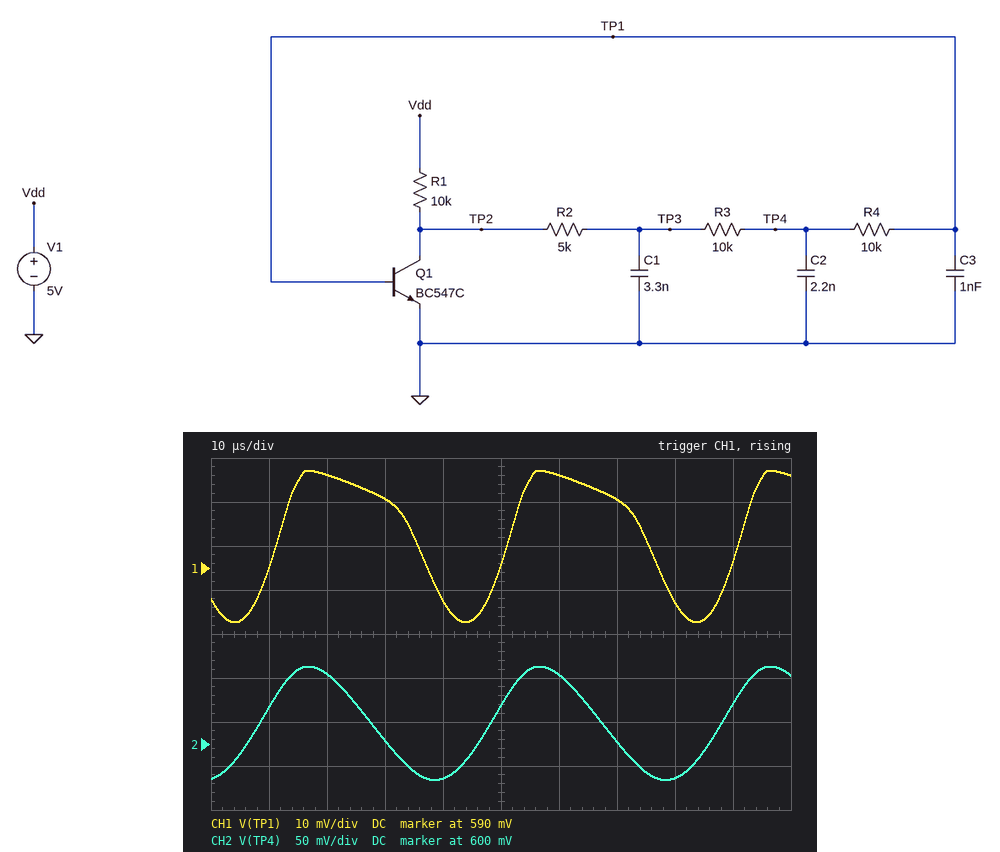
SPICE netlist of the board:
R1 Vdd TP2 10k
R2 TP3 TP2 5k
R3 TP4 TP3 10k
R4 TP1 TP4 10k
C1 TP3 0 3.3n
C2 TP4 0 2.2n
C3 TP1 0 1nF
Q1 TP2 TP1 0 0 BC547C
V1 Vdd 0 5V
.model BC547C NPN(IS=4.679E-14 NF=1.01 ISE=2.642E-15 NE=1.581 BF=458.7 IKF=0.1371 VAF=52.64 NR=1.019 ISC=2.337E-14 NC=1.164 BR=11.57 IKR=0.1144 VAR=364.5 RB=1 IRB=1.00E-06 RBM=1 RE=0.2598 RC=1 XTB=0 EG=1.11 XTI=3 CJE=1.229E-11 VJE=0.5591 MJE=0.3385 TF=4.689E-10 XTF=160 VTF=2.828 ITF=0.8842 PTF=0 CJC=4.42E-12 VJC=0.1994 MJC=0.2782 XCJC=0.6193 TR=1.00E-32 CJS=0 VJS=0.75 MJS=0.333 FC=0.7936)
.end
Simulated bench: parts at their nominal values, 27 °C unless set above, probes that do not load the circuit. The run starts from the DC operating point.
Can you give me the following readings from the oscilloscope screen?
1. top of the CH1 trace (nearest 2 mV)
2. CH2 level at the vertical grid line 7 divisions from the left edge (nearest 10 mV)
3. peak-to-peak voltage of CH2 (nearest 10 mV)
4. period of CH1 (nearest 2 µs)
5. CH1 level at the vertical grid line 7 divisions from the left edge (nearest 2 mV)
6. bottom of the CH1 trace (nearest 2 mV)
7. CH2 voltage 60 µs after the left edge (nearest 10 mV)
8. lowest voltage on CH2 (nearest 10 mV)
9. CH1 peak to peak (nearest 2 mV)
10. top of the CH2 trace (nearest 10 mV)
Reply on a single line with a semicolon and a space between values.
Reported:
612 mV; 600 mV; 130 mV; 40 µs; 606 mV; 578 mV; 680 mV; 560 mV; 34 mV; 690 mV
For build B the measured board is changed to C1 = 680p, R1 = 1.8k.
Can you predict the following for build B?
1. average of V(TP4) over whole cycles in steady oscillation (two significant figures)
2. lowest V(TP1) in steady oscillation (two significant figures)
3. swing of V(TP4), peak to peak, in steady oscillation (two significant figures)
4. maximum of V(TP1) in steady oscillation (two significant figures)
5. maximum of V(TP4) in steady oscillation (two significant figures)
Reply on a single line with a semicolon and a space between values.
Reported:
700 mV; 640 mV; 100 mV; 650 mV; 750 mV
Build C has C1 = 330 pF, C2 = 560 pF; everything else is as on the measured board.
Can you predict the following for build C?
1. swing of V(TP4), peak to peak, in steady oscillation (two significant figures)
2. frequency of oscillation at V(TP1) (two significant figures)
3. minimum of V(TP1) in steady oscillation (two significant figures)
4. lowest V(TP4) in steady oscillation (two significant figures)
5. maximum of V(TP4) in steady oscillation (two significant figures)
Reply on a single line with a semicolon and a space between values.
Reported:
210 mV; 91 kHz; 590 mV; 520 mV; 730 mV
